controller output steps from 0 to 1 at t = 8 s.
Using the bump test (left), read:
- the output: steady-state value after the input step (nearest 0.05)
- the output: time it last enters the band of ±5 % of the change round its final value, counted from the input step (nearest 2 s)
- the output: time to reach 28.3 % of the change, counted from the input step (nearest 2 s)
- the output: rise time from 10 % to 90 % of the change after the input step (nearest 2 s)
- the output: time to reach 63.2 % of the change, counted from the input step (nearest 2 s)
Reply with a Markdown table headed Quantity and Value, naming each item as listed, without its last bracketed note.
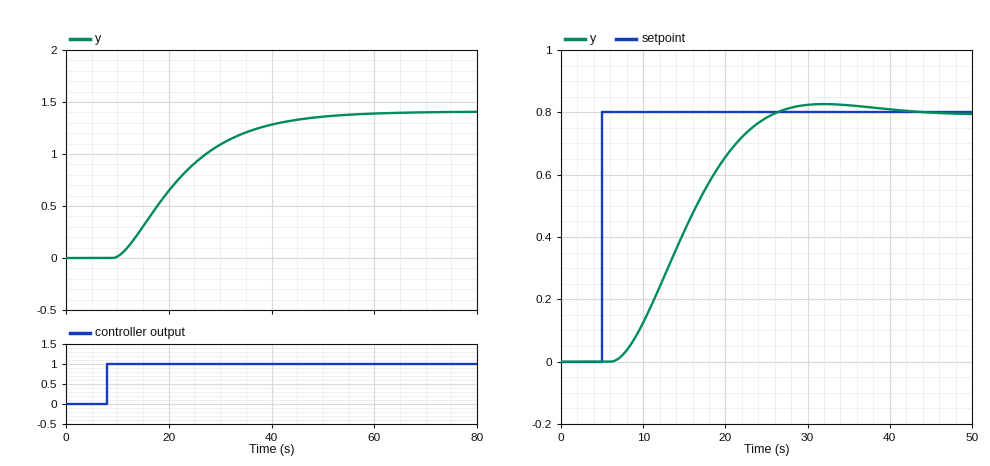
| Quantity | Value |
|---|---|
| the output: steady-state value after the input step | 1.40 |
| the output: time it last enters the band of ±5 % of the change round its final value, counted from the input step | 38 s |
| the output: time to reach 28.3 % of the change, counted from the input step | 8 s |
| the output: rise time from 10 % to 90 % of the change after the input step | 26 s |
| the output: time to reach 63.2 % of the change, counted from the input step | 16 s |
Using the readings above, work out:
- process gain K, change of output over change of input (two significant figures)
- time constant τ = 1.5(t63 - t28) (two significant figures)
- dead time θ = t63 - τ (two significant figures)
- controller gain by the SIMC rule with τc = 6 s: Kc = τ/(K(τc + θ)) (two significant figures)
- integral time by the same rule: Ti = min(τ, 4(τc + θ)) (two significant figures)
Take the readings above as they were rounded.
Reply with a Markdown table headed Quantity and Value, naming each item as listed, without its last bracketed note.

| Quantity | Value |
|---|---|
| process gain K, change of output over change of input | 1.4 |
| time constant τ = 1.5(t63 - t28) | 12 s |
| dead time θ = t63 - τ | 4.0 s |
| controller gain by the SIMC rule with τc = 6 s: Kc = τ/(K(τc + θ)) | 0.86 |
| integral time by the same rule: Ti = min(τ, 4(τc + θ)) | 12 s |
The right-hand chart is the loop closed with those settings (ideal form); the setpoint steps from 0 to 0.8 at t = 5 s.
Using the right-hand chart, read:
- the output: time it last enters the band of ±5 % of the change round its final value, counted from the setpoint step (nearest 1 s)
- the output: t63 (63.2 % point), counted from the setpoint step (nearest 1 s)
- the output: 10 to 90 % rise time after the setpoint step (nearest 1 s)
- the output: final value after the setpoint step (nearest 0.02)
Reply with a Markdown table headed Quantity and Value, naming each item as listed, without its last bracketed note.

| Quantity | Value |
|---|---|
| the output: time it last enters the band of ±5 % of the change round its final value, counted from the setpoint step | 19 s |
| the output: t63 (63.2 % point), counted from the setpoint step | 12 s |
| the output: 10 to 90 % rise time after the setpoint step | 13 s |
| the output: final value after the setpoint step | 0.80 |
